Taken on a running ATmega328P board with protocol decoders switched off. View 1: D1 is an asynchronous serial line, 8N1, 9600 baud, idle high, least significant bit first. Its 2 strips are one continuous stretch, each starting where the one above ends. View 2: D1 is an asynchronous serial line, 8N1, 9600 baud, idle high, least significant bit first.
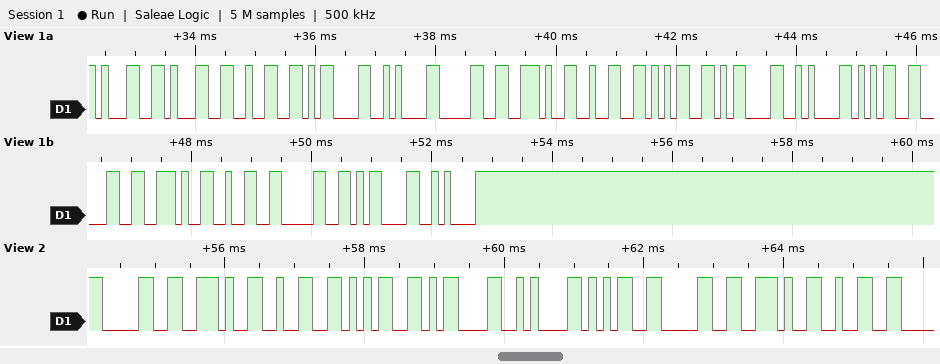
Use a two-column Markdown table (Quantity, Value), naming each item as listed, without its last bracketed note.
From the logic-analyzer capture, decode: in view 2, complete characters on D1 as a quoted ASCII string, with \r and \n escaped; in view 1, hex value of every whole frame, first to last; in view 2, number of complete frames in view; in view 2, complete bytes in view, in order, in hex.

| Quantity | Value |
|---|---|
| in view 2, complete characters on D1 as a quoted ASCII string, with \r and \n escaped | "0.25\r\n50.2" |
| in view 1, hex value of every whole frame, first to last | 0x31 0x31 0x32 0x0D 0x0A 0x30 0x2E 0x32 0x35 0x0D 0x0A 0x35 0x30 0x2E 0x32 0x30 0x0D 0x0A |
| in view 2, number of complete frames in view | 10 |
| in view 2, complete bytes in view, in order, in hex | 30 2E 32 35 0D 0A 35 30 2E 32 |
